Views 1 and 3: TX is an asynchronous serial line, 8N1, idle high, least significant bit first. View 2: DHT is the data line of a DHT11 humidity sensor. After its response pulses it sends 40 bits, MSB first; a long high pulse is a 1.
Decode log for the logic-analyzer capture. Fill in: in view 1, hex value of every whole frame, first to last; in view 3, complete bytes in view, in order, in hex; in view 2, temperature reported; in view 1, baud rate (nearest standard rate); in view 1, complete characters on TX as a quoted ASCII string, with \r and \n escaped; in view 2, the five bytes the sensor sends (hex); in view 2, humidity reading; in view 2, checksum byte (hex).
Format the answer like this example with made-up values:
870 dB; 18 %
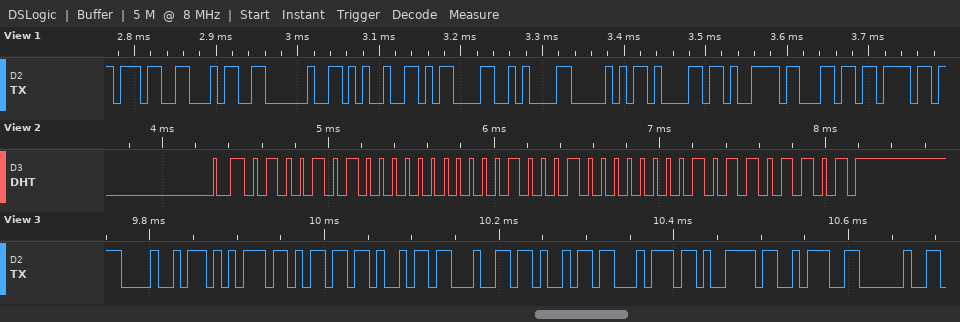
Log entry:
0x37 0x34 0x20 0x25 0x0D 0x0A 0x50 0x61 0x79 0x6C 0x6F; 48 75 6D 69 64 69 74 79 3A 20; 34.1 °C; 115200 baud; "74 %\r\nPaylo"; 4A 00 22 01 6D; 74 %; 0x6D
